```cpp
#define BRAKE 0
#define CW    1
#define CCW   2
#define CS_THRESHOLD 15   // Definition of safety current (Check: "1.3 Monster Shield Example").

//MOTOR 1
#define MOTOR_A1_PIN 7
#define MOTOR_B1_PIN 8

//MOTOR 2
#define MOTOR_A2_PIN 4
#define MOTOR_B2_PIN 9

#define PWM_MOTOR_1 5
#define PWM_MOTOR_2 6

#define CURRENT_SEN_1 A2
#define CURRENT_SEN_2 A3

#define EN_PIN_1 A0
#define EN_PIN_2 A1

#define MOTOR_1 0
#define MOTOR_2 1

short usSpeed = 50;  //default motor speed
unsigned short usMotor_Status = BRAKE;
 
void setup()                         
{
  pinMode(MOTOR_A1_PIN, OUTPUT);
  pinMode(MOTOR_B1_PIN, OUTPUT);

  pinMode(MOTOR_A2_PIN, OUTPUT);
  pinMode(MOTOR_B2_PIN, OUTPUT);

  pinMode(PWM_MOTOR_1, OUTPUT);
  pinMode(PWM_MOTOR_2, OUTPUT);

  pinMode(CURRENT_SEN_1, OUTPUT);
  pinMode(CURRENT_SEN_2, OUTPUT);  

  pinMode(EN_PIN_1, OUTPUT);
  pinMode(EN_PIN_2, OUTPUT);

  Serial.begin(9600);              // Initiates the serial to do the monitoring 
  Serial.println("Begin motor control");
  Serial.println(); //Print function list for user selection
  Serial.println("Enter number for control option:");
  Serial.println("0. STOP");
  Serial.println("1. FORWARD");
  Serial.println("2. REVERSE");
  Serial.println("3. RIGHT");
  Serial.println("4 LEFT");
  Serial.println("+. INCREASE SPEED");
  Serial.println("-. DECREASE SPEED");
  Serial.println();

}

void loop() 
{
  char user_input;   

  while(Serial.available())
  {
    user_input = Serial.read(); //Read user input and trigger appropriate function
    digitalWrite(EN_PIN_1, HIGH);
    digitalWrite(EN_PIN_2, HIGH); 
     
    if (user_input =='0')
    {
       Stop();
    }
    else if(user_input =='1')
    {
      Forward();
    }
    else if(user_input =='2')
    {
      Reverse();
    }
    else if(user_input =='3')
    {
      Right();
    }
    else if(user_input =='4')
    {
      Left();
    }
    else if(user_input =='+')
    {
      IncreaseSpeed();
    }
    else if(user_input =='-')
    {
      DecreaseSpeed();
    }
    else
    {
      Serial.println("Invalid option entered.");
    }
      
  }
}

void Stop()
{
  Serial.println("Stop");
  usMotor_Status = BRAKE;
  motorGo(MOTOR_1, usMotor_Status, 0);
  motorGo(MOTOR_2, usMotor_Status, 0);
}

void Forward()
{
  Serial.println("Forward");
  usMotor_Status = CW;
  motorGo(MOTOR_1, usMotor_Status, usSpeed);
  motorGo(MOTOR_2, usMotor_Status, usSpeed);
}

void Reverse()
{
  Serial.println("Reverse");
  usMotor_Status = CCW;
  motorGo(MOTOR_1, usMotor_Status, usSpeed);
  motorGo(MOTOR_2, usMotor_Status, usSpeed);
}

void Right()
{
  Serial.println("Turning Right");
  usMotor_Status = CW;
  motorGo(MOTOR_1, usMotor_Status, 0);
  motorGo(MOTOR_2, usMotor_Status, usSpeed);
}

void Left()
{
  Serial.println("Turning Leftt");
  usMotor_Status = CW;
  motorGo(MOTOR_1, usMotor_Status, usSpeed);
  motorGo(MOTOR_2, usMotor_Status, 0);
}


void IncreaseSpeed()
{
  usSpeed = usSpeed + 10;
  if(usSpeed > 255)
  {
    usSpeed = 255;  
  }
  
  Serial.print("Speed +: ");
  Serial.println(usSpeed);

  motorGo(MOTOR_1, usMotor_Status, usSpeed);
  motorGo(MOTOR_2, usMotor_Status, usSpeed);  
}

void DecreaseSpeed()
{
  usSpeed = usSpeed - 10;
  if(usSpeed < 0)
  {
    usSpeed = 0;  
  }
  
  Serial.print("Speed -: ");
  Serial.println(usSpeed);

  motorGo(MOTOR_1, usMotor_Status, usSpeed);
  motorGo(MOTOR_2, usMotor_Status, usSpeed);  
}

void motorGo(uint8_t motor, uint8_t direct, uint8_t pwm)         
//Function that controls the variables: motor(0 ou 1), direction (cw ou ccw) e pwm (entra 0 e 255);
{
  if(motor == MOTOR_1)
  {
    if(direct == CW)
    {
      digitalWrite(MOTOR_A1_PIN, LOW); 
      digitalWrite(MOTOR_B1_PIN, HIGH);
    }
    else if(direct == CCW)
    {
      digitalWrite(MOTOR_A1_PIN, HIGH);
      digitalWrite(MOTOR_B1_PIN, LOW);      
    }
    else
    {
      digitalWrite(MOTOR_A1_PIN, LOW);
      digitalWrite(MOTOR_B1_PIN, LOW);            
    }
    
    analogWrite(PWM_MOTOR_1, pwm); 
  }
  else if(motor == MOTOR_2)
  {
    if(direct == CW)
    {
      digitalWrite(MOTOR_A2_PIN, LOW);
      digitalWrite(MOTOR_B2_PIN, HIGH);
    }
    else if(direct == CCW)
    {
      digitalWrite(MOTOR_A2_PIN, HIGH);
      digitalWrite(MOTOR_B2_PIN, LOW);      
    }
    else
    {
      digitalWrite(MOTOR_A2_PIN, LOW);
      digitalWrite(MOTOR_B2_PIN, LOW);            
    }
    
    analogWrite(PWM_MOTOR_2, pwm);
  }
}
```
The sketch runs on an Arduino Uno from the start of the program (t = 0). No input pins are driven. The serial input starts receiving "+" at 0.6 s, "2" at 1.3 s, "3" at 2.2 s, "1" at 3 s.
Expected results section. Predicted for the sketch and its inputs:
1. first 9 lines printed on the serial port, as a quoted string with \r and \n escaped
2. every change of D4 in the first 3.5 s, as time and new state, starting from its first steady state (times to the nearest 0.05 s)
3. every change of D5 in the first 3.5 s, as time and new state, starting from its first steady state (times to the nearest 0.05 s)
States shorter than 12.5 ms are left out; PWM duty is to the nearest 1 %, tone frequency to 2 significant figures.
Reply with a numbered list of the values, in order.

1. "Begin motor control\r\n\r\nEnter number for control option:\r\n0. STOP\r\n1. FORWARD\r\n2. REVERSE\r\n3. RIGHT\r\n4 LEFT\r\n+. INCREASE SPEED\r\n"
2. 0 s low; 1.3 s high; 2.2 s low
3. 0 s low; 0.6 s PWM 24 %; 2.2 s low; 3 s PWM 24 %
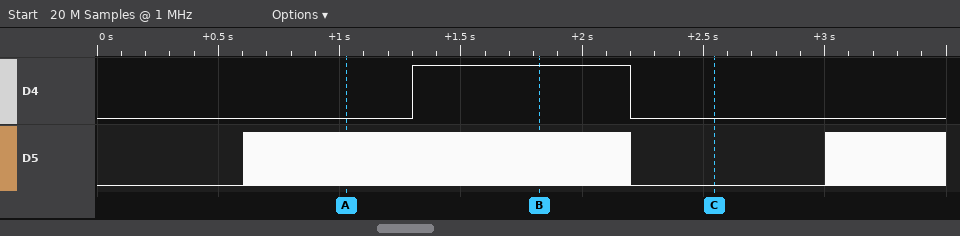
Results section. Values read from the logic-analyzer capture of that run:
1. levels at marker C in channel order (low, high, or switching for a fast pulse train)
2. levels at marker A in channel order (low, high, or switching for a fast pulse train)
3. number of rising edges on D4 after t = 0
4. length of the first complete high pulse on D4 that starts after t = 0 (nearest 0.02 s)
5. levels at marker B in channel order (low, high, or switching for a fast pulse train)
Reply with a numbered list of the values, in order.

1. D4 low, D5 low
2. D4 low, D5 switching
3. 1
4. 0.90 s
5. D4 high, D5 switching
